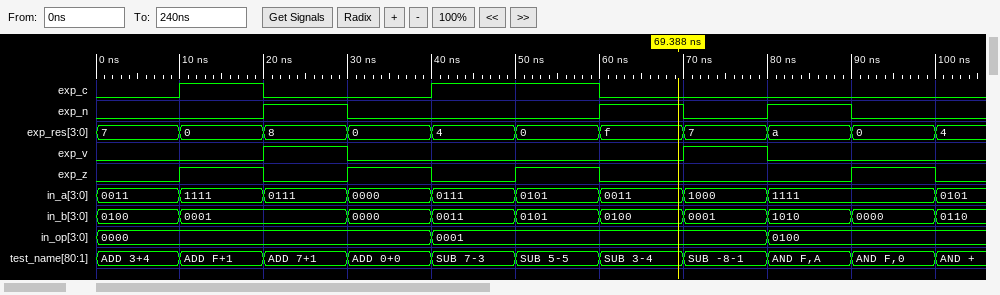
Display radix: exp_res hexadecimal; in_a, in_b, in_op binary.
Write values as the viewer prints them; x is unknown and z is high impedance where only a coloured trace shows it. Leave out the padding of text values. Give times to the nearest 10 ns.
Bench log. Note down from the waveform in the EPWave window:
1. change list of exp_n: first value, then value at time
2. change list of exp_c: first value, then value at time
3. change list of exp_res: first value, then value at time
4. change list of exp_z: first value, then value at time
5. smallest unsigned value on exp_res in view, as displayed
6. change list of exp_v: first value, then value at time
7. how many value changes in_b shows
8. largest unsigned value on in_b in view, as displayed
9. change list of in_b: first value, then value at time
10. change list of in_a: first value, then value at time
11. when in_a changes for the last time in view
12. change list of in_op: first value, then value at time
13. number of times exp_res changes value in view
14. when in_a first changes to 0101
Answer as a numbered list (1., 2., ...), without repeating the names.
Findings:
1. 0, 1 at 20 ns, 0 at 30 ns, 1 at 60 ns, 0 at 70 ns, 1 at 80 ns, 0 at 90 ns
2. 0, 1 at 10 ns, 0 at 20 ns, 1 at 40 ns, 0 at 60 ns
3. 7, 0 at 10 ns, 8 at 20 ns, 0 at 30 ns, 4 at 40 ns, 0 at 50 ns, f at 60 ns, 7 at 70 ns, a at 80 ns, 0 at 90 ns, 4 at 100 ns
4. 0, 1 at 10 ns, 0 at 20 ns, 1 at 30 ns, 0 at 40 ns, 1 at 50 ns, 0 at 60 ns, 1 at 90 ns, 0 at 100 ns
5. 0
6. 0, 1 at 20 ns, 0 at 30 ns, 1 at 70 ns, 0 at 80 ns
7. 9
8. 1010
9. 0100, 0001 at 10 ns, 0000 at 30 ns, 0011 at 40 ns, 0101 at 50 ns, 0100 at 60 ns, 0001 at 70 ns, 1010 at 80 ns, 0000 at 90 ns, 0110 at 100 ns
10. 0011, 1111 at 10 ns, 0111 at 20 ns, 0000 at 30 ns, 0111 at 40 ns, 0101 at 50 ns, 0011 at 60 ns, 1000 at 70 ns, 1111 at 80 ns, 0101 at 100 ns
11. 100 ns
12. 0000, 0001 at 40 ns, 0100 at 80 ns
13. 10
14. 50 ns
